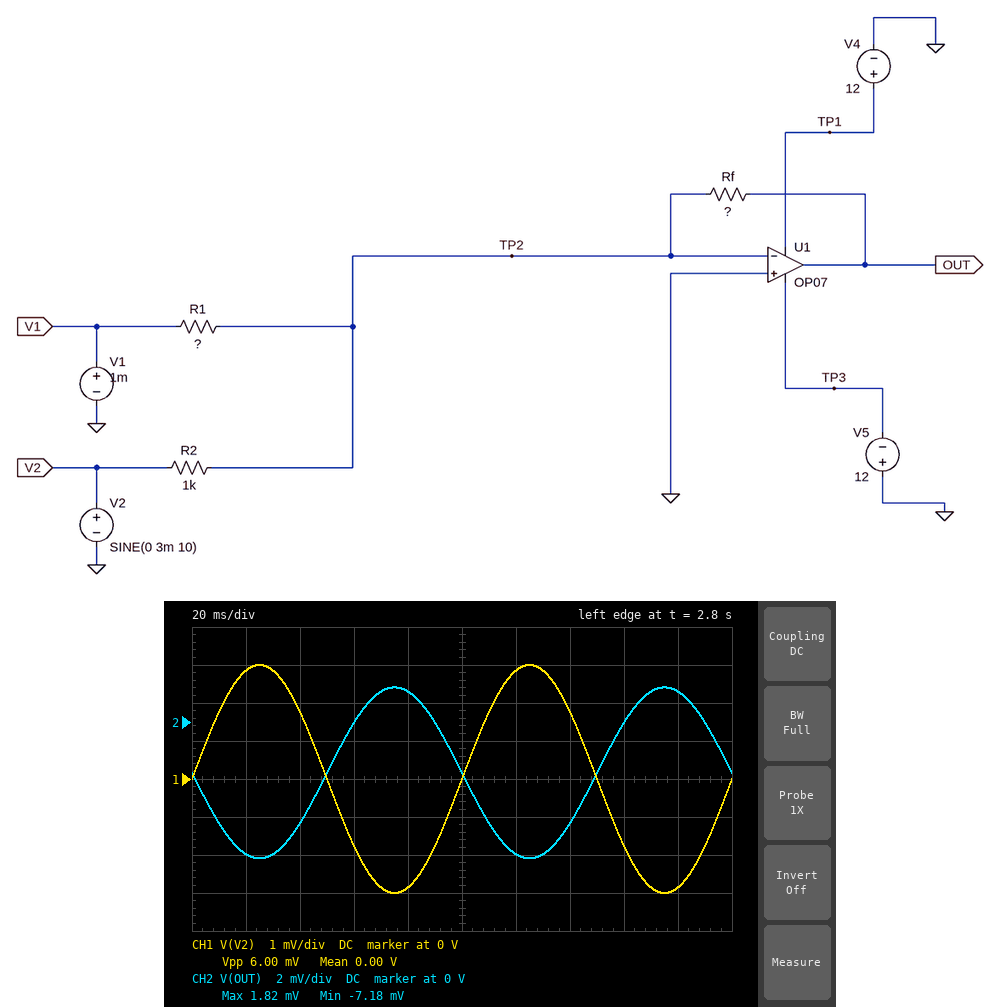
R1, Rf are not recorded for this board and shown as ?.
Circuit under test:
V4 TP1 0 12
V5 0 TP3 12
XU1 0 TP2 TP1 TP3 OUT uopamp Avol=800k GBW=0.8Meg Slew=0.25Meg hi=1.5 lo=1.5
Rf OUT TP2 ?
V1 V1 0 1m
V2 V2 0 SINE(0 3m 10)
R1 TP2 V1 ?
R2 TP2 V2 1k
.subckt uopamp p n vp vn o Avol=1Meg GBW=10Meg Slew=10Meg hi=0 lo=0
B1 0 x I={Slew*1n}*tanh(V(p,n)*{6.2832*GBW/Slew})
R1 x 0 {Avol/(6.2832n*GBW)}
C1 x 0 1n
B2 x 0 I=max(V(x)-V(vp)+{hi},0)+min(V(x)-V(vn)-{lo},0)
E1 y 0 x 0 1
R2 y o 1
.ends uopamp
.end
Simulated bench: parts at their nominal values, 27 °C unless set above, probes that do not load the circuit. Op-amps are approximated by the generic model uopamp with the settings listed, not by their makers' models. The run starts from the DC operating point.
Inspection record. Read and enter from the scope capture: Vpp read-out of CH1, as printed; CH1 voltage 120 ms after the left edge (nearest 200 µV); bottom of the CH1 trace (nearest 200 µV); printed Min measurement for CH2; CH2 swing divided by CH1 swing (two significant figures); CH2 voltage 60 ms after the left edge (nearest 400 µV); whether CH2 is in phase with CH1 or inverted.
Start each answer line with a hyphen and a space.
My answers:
- 6.00 mV
- 2.8 mV
- -3.0 mV
- -7.18 mV
- 1.5
- 0 V
- inverted
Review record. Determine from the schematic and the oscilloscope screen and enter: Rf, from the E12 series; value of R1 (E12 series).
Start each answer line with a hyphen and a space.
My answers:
- 1.5 kΩ
- 560 Ω
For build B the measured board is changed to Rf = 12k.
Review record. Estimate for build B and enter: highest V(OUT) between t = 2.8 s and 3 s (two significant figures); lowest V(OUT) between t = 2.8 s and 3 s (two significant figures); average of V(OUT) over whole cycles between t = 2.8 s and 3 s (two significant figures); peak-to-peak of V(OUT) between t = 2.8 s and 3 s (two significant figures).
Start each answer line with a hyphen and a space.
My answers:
- 15 mV
- -57 mV
- -21 mV
- 72 mV
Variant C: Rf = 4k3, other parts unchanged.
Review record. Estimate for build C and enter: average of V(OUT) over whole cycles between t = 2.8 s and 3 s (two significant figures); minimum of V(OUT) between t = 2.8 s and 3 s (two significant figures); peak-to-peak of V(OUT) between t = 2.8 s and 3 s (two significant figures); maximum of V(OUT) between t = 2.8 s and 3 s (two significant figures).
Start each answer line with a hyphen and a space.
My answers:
- -7.7 mV
- -21 mV
- 26 mV
- 5.2 mV
